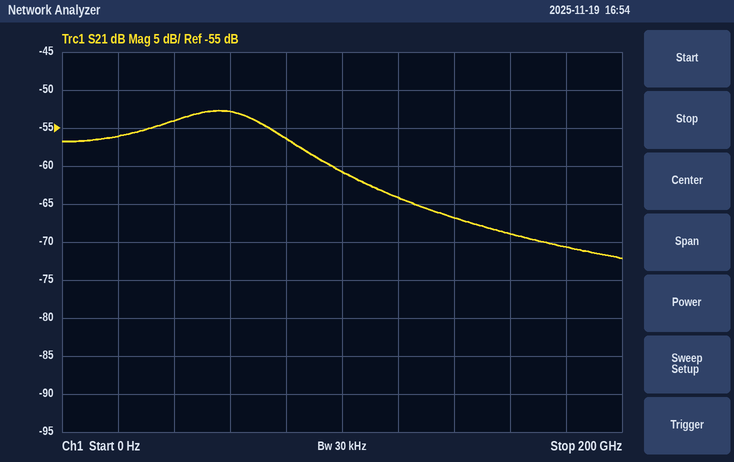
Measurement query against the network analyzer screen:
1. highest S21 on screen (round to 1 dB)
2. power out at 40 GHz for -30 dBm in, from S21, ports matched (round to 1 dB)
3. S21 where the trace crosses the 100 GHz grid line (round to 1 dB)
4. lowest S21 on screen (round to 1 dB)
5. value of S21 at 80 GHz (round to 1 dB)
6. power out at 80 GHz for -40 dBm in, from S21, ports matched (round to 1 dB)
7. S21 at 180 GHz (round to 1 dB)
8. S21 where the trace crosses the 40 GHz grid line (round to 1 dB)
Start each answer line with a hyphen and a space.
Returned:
- -53 dB
- -84 dBm
- -61 dB
- -72 dB
- -56 dB
- -96 dBm
- -71 dB
- -54 dB
